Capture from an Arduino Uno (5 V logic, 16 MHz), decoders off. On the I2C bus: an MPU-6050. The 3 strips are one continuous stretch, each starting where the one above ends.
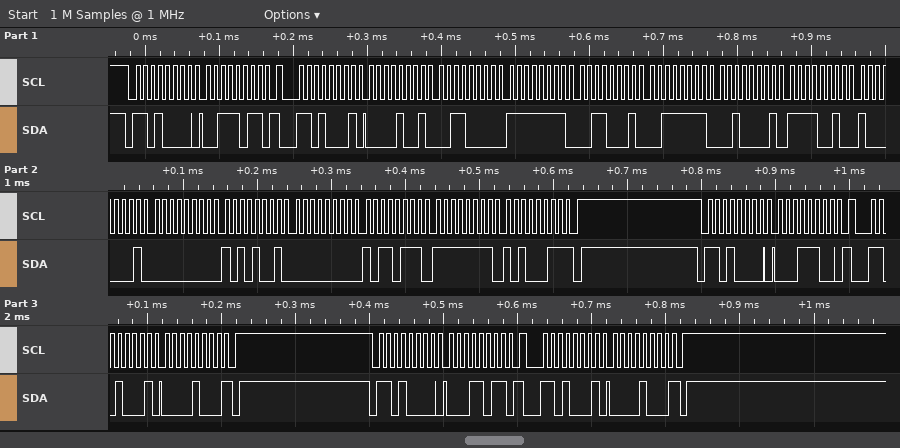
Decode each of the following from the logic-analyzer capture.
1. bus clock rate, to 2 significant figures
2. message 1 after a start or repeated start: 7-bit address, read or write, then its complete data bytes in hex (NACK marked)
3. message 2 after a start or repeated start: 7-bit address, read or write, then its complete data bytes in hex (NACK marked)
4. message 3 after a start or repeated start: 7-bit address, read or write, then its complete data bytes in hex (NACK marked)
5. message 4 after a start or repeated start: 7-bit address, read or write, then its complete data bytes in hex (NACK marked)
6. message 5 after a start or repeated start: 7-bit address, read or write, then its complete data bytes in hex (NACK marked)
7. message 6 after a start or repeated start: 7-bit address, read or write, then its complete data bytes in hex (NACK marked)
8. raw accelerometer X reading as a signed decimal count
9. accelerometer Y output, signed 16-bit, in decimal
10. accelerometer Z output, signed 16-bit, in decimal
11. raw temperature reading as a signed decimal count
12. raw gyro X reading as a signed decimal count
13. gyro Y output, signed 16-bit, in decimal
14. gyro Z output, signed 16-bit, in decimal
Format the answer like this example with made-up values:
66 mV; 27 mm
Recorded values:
100 kHz; 0x68 write: 3B; 0x68 read: 09 30 FF 31 3F 21 F2 81 00 A9 00 B7 FF A3 NACK; 0x68 write: 1C; 0x68 read: 08 NACK; 0x68 write: 1B; 0x68 read: 08 NACK; 2352; -207; 16161; -3455; 169; 183; -93
